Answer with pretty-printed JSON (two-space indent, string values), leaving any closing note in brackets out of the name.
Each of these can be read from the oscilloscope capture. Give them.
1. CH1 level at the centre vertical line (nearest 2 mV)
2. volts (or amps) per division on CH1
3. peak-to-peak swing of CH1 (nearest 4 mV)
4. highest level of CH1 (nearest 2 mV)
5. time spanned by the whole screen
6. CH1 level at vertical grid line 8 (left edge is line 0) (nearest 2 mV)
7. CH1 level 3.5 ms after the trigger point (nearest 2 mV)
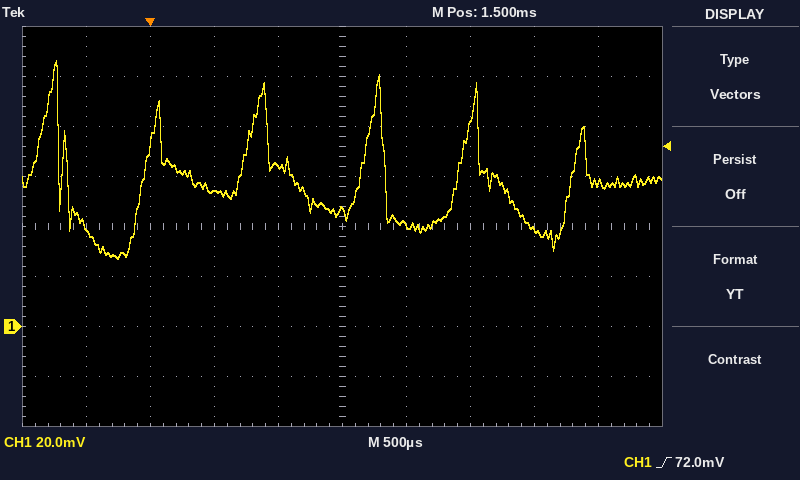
{
  "CH1 level at the centre vertical line": "46 mV",
  "volts (or amps) per division on CH1": "20 mV",
  "peak-to-peak swing of CH1": "80 mV",
  "highest level of CH1": "106 mV",
  "time spanned by the whole screen": "5 ms",
  "CH1 level at vertical grid line 8 (left edge is line 0)": "38 mV",
  "CH1 level 3.5 ms after the trigger point": "58 mV"
}
